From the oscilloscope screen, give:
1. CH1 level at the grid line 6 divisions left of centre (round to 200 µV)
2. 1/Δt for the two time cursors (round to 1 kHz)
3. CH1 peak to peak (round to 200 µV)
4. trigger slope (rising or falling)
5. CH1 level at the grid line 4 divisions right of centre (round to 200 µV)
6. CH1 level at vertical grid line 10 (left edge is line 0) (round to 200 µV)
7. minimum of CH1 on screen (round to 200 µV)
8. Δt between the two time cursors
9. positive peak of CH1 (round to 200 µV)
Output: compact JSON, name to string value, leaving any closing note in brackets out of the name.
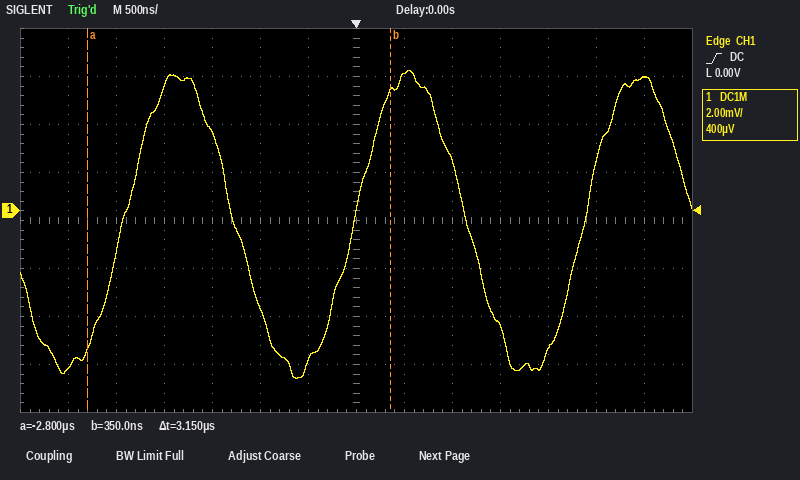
{"CH1 level at the grid line 6 divisions left of centre": "-6.6 mV", "1/Δt for the two time cursors": "317 kHz", "CH1 peak to peak": "12.8 mV", "trigger slope": "rising", "CH1 level at the grid line 4 divisions right of centre": "-5.8 mV", "CH1 level at vertical grid line 10 (left edge is line 0)": "-4.8 mV", "minimum of CH1 on screen": "-7.0 mV", "Δt between the two time cursors": "3.15 µs", "positive peak of CH1": "5.8 mV"}
